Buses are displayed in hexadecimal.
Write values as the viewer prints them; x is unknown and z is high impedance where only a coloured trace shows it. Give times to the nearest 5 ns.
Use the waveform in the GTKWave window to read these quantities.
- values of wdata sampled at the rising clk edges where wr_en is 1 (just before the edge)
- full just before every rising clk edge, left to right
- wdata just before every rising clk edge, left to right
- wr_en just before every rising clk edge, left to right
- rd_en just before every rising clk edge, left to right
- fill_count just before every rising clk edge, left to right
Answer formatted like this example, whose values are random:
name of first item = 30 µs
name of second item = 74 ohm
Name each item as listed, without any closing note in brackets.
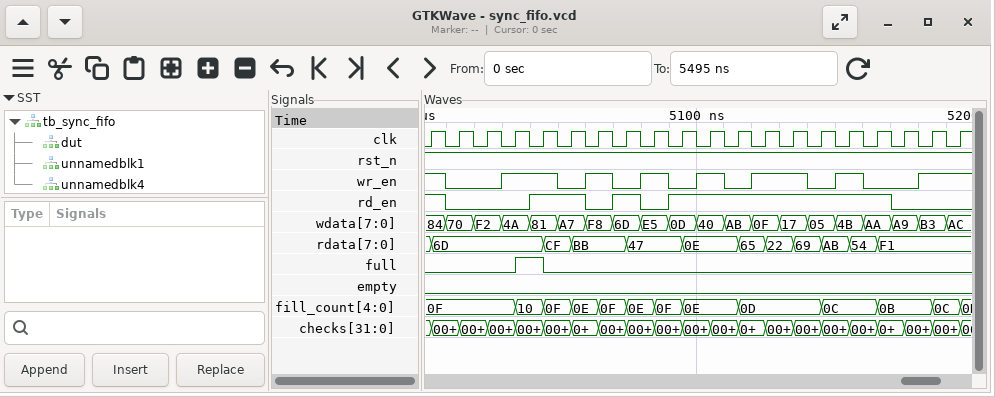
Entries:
values of wdata sampled at the rising clk edges where wr_en is 1 = 84, 4A, 81, F8, E5, 40, 0F, 17, 4B, B3, AC
full just before every rising clk edge, left to right = 0 0 0 0 1 0 0 0 0 0 0 0 0 0 0 0 0 0 0 0
wdata just before every rising clk edge, left to right = 84, 70, F2, 4A, 81, A7, F8, 6D, E5, 0D, 40, AB, 0F, 17, 05, 4B, AA, A9, B3, AC
wr_en just before every rising clk edge, left to right = 1 0 0 1 1 0 1 0 1 0 1 0 1 1 0 1 0 0 1 1
rd_en just before every rising clk edge, left to right = 1 0 0 0 1 1 0 1 0 1 1 1 1 1 1 1 1 0 0 0
fill_count just before every rising clk edge, left to right = 0F, 0F, 0F, 0F, 10, 0F, 0E, 0F, 0E, 0F, 0E, 0E, 0D, 0D, 0D, 0C, 0C, 0B, 0B, 0C
